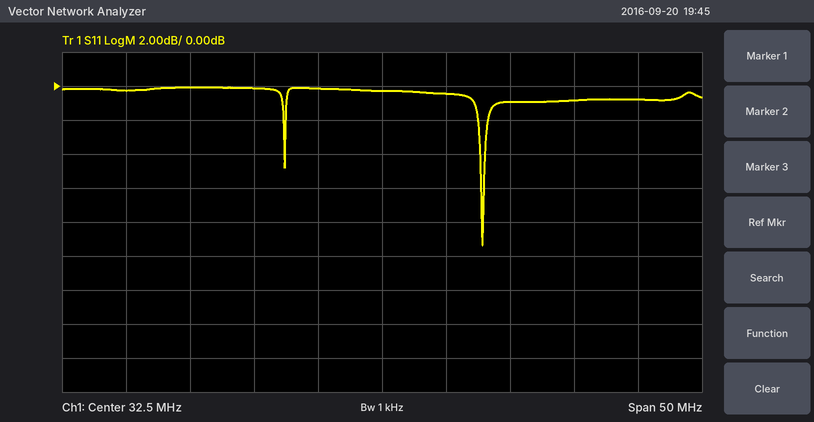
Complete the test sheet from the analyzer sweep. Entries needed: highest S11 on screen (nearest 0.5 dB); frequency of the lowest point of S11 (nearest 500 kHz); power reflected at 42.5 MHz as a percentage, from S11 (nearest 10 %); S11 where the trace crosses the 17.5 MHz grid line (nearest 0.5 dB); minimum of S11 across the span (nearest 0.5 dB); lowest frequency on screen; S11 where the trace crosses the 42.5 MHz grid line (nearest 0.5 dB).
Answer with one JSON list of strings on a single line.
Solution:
["0.0 dB", "40.5 MHz", "80 %", "0.0 dB", "-9.5 dB", "7.5 MHz", "-1.0 dB"]
